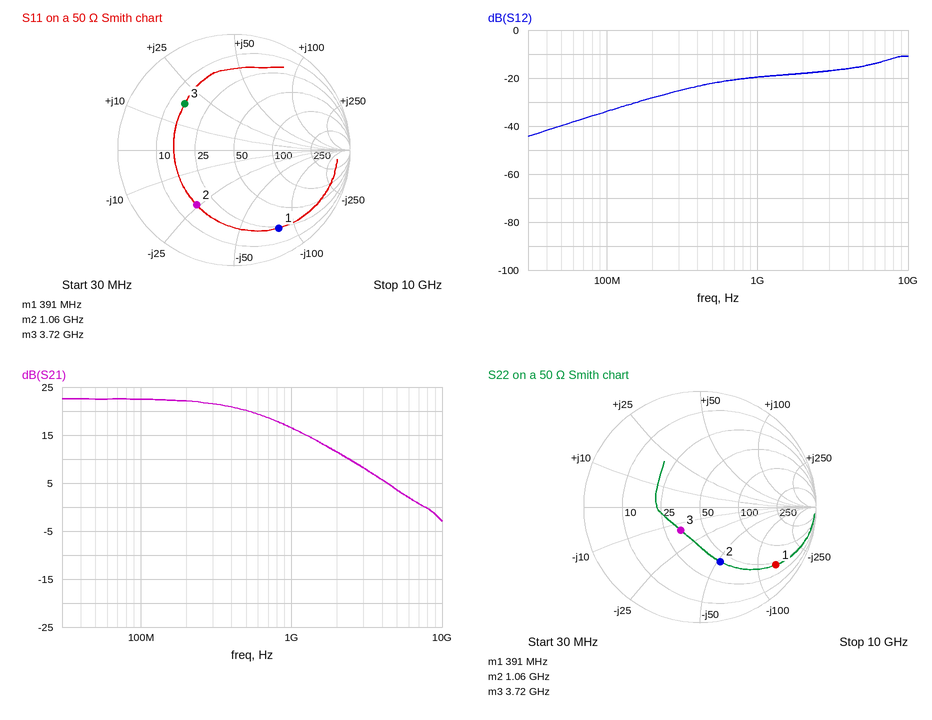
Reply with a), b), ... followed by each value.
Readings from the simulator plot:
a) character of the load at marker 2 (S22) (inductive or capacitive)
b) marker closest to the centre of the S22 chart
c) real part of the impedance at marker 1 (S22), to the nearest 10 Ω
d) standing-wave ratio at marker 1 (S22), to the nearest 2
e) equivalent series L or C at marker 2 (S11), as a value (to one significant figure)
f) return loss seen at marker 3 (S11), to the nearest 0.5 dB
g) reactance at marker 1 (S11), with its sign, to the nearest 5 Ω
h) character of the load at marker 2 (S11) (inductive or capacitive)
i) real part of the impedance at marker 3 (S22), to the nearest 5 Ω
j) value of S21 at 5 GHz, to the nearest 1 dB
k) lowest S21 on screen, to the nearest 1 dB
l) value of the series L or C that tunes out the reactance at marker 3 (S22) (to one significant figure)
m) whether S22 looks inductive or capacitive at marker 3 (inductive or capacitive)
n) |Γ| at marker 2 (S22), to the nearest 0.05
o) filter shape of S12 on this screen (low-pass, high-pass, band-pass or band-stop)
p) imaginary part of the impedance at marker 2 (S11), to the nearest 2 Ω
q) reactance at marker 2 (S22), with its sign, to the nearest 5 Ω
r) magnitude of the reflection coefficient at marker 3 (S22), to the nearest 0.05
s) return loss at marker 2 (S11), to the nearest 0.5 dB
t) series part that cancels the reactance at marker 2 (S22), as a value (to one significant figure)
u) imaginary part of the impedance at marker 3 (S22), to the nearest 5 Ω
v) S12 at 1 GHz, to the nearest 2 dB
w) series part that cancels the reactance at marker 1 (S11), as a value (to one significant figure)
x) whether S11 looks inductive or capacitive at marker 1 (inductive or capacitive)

a) capacitive
b) marker 3
c) 40 Ω
d) 10
e) 6 pF
f) 4.5 dB
g) -80 Ω
h) capacitive
i) 35 Ω
j) 4 dB
k) -3 dB
l) 600 pH
m) capacitive
n) 0.50
o) high-pass
p) -24 Ω
q) -50 Ω
r) 0.25
s) 5.0 dB
t) 8 nH
u) -15 Ω
v) -20 dB
w) 30 nH
x) capacitive
